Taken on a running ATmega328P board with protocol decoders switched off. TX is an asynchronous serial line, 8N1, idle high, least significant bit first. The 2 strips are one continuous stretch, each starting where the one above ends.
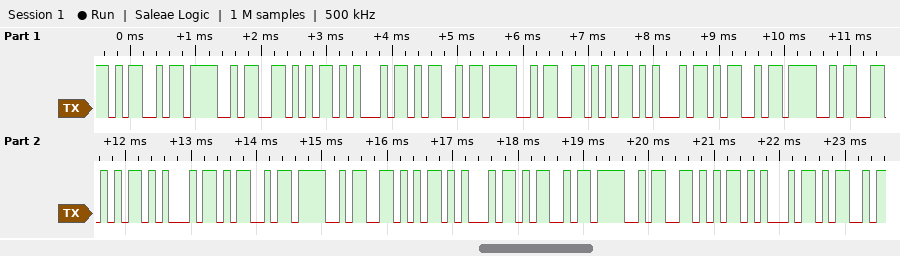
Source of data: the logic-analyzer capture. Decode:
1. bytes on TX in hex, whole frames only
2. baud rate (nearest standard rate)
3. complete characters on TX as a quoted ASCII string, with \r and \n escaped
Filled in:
4D 4F 56 45 4D 4F 56 45 4D 4F 56 45 4D 4F 56 45 4D 4F 56 45 4D
9600 baud
"MOVEMOVEMOVEMOVEMOVEM"
